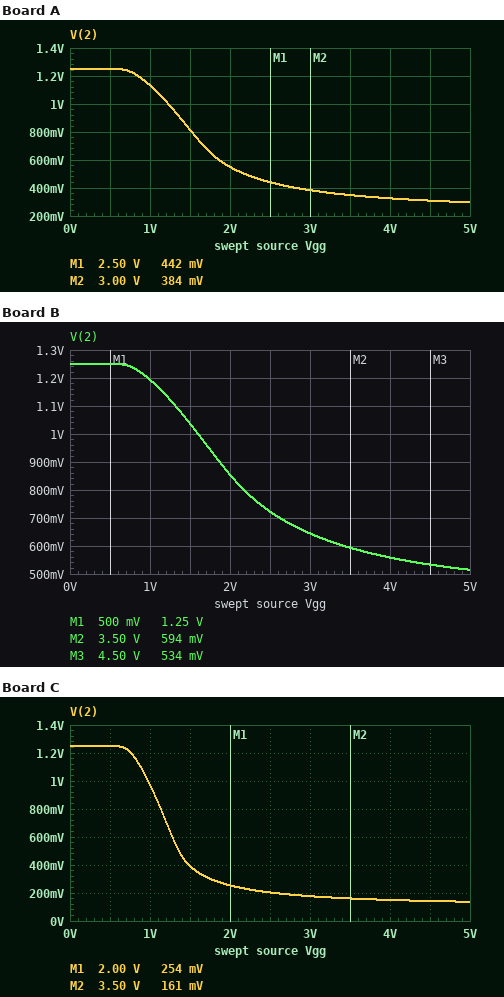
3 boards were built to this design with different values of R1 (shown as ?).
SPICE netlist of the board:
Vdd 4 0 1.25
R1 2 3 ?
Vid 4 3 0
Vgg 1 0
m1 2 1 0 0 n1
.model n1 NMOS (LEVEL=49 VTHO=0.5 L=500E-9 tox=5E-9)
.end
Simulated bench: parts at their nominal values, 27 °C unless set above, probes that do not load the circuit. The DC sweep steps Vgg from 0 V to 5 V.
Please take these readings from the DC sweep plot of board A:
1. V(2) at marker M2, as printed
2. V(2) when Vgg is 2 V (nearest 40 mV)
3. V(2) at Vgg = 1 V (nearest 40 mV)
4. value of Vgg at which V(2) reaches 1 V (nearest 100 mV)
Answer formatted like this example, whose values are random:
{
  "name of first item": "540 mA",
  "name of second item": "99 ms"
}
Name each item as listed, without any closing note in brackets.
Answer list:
{
  "V(2) at marker M2, as printed": "384 mV",
  "V(2) when Vgg is 2 V": "560 mV",
  "V(2) at Vgg = 1 V": "1.12 V",
  "value of Vgg at which V(2) reaches 1 V": "1.2 V"
}
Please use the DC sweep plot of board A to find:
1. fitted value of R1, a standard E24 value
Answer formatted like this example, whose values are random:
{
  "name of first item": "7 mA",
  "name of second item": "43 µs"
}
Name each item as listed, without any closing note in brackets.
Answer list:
{
  "fitted value of R1, a standard E24 value": "750 Ω"
}
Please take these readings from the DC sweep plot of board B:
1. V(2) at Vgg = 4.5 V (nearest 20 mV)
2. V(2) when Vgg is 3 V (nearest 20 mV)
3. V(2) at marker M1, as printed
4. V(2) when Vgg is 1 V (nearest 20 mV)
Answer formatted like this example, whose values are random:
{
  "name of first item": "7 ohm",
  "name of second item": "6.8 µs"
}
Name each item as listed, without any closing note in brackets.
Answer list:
{
  "V(2) at Vgg = 4.5 V": "540 mV",
  "V(2) when Vgg is 3 V": "640 mV",
  "V(2) at marker M1, as printed": "1.25 V",
  "V(2) when Vgg is 1 V": "1.20 V"
}
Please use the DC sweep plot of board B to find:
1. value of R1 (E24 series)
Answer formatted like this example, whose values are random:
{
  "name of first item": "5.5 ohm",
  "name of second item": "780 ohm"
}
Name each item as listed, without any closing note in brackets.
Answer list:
{
  "value of R1": "360 Ω"
}
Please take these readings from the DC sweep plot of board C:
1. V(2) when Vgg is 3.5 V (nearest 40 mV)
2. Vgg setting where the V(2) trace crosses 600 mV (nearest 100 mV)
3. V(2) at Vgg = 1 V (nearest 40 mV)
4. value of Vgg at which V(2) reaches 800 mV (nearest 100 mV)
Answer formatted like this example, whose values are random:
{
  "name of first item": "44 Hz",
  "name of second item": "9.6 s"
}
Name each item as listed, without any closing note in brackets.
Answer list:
{
  "V(2) when Vgg is 3.5 V": "160 mV",
  "Vgg setting where the V(2) trace crosses 600 mV": "1.3 V",
  "V(2) at Vgg = 1 V": "960 mV",
  "value of Vgg at which V(2) reaches 800 mV": "1.1 V"
}
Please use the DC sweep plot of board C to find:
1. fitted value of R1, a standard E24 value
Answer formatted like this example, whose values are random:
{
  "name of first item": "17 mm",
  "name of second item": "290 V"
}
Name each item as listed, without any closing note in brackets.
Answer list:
{
  "fitted value of R1, a standard E24 value": "1.8 kΩ"
}
